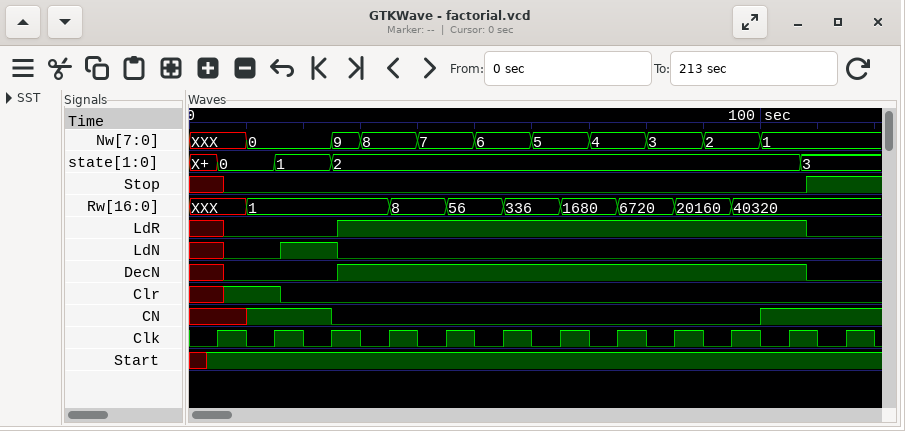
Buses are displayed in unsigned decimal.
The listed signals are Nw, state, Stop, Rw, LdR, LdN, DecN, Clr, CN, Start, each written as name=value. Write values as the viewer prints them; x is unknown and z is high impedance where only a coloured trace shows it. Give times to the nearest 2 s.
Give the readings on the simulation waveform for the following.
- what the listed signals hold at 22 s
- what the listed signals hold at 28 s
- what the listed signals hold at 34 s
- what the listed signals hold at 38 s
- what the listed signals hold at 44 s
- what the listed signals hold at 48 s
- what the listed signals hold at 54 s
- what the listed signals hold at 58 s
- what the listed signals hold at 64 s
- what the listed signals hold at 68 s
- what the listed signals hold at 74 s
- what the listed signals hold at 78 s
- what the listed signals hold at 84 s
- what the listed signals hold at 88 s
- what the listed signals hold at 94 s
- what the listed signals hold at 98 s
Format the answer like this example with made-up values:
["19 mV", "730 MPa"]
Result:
["Nw=0, state=1, Stop=0, Rw=1, LdR=0, LdN=1, DecN=0, Clr=0, CN=1, Start=1", "Nw=9, state=2, Stop=0, Rw=1, LdR=1, LdN=0, DecN=1, Clr=0, CN=0, Start=1", "Nw=8, state=2, Stop=0, Rw=1, LdR=1, LdN=0, DecN=1, Clr=0, CN=0, Start=1", "Nw=8, state=2, Stop=0, Rw=8, LdR=1, LdN=0, DecN=1, Clr=0, CN=0, Start=1", "Nw=7, state=2, Stop=0, Rw=8, LdR=1, LdN=0, DecN=1, Clr=0, CN=0, Start=1", "Nw=7, state=2, Stop=0, Rw=56, LdR=1, LdN=0, DecN=1, Clr=0, CN=0, Start=1", "Nw=6, state=2, Stop=0, Rw=56, LdR=1, LdN=0, DecN=1, Clr=0, CN=0, Start=1", "Nw=6, state=2, Stop=0, Rw=336, LdR=1, LdN=0, DecN=1, Clr=0, CN=0, Start=1", "Nw=5, state=2, Stop=0, Rw=336, LdR=1, LdN=0, DecN=1, Clr=0, CN=0, Start=1", "Nw=5, state=2, Stop=0, Rw=1680, LdR=1, LdN=0, DecN=1, Clr=0, CN=0, Start=1", "Nw=4, state=2, Stop=0, Rw=1680, LdR=1, LdN=0, DecN=1, Clr=0, CN=0, Start=1", "Nw=4, state=2, Stop=0, Rw=6720, LdR=1, LdN=0, DecN=1, Clr=0, CN=0, Start=1", "Nw=3, state=2, Stop=0, Rw=6720, LdR=1, LdN=0, DecN=1, Clr=0, CN=0, Start=1", "Nw=3, state=2, Stop=0, Rw=20160, LdR=1, LdN=0, DecN=1, Clr=0, CN=0, Start=1", "Nw=2, state=2, Stop=0, Rw=20160, LdR=1, LdN=0, DecN=1, Clr=0, CN=0, Start=1", "Nw=2, state=2, Stop=0, Rw=40320, LdR=1, LdN=0, DecN=1, Clr=0, CN=0, Start=1"]
